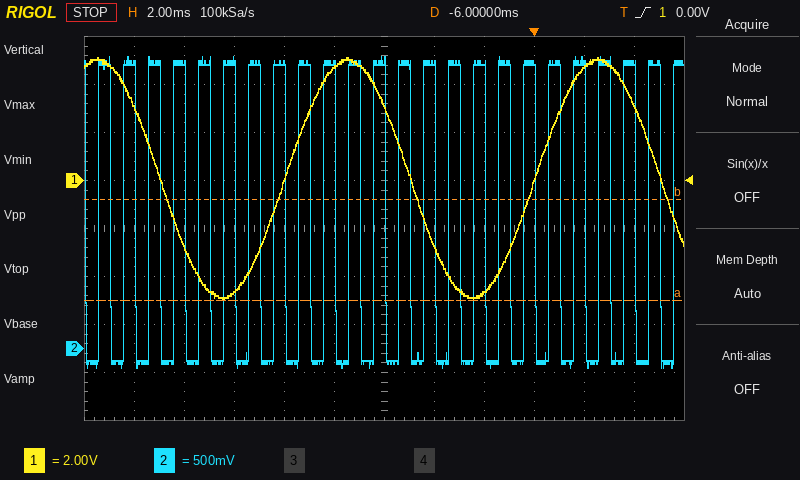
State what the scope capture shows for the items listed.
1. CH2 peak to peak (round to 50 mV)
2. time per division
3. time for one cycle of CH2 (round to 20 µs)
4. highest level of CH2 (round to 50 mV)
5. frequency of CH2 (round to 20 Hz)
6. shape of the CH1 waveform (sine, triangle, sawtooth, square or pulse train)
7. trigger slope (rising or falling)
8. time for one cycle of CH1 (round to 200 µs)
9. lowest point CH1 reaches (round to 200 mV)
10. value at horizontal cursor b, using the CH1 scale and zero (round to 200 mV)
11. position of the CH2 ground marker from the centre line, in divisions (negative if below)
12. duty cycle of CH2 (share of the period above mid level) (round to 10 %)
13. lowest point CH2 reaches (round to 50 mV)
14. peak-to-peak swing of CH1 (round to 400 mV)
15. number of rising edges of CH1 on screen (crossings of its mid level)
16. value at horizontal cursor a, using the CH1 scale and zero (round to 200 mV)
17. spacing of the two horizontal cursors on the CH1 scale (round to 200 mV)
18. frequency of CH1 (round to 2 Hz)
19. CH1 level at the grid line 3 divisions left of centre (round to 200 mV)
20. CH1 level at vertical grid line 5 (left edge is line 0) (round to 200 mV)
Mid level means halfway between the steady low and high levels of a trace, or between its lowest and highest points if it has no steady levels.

3.25 V
2 ms
1.00 ms
3.05 V
1.00 kHz
sine
rising
10.0 ms
-5.0 V
-800 mV
-2.5 div
50 %
-200 mV
10.0 V
2
-5.0 V
4.2 V
100 Hz
-4.6 V
4.6 V
